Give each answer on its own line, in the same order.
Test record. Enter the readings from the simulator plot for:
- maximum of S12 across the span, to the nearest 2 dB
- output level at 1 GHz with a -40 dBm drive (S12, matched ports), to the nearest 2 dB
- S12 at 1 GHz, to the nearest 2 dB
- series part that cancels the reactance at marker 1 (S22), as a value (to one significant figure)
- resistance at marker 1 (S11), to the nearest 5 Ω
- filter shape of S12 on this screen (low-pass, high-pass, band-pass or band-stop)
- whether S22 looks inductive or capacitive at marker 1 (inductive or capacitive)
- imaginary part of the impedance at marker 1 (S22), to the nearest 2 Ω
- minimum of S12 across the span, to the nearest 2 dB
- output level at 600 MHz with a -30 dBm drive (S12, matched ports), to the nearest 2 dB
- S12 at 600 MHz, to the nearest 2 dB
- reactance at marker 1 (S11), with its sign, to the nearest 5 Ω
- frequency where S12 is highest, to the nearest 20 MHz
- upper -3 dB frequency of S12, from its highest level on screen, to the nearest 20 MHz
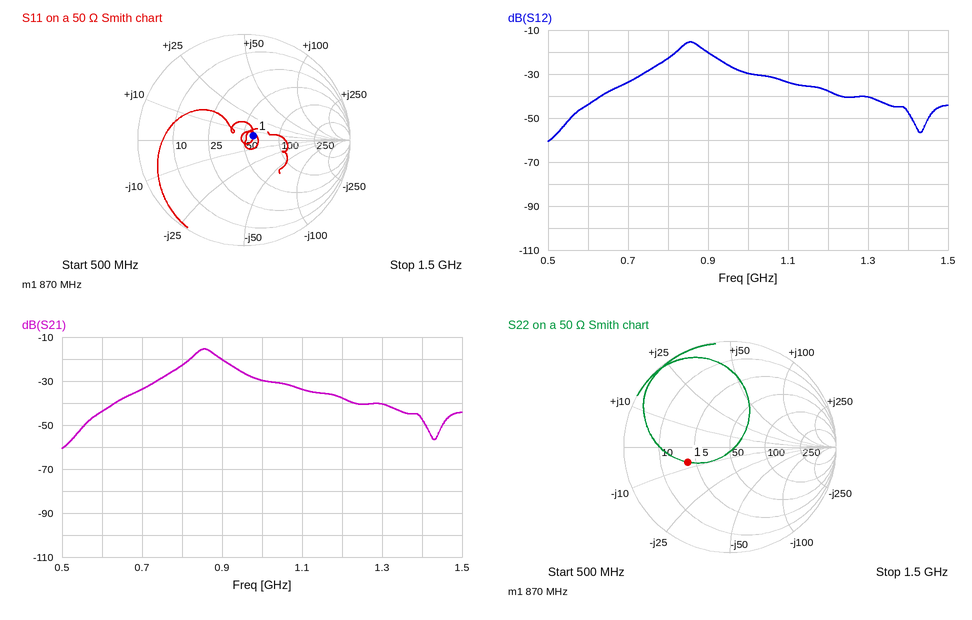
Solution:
-16 dB
-70 dBm
-30 dB
1 nH
60 Ω
band-pass
capacitive
-8 Ω
-60 dB
-74 dBm
-44 dB
+5 Ω
860 MHz
880 MHz
